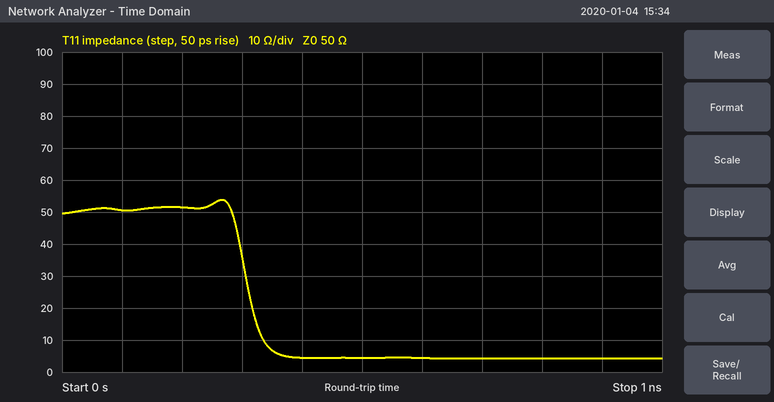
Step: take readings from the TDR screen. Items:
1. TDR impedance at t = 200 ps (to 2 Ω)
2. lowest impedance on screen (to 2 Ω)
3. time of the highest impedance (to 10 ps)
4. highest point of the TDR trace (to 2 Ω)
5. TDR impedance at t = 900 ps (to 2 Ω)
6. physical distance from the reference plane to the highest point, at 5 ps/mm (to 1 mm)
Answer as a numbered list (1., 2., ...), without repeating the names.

1. 52 Ω
2. 4 Ω
3. 270 ps
4. 54 Ω
5. 4 Ω
6. 27 mm
